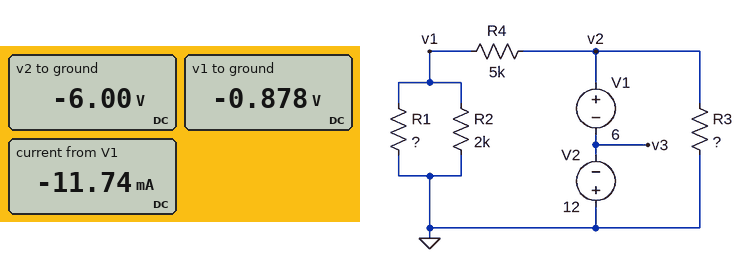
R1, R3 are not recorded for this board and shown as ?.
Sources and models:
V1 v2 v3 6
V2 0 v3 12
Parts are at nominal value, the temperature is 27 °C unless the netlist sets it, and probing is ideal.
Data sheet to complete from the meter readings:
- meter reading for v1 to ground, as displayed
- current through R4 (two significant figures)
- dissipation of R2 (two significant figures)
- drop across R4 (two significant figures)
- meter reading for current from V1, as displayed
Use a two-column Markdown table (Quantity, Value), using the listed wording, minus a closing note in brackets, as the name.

| Quantity | Value |
|---|---|
| meter reading for v1 to ground, as displayed | -0.878 V |
| current through R4 | 1.0 mA |
| dissipation of R2 | 390 µW |
| drop across R4 | 5.1 V |
| meter reading for current from V1, as displayed | -11.74 mA |
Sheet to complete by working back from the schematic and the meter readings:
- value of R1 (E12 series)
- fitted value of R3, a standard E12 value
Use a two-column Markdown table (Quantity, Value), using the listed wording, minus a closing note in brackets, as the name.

| Quantity | Value |
|---|---|
| value of R1 | 1.5 kΩ |
| fitted value of R3, a standard E12 value | 560 Ω |
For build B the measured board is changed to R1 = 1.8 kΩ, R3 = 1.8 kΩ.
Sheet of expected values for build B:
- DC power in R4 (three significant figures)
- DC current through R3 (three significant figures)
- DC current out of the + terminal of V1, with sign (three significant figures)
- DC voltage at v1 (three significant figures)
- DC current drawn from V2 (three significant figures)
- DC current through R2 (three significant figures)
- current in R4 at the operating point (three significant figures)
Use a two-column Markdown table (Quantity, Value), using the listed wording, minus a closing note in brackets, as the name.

| Quantity | Value |
|---|---|
| DC power in R4 | 5.09 mW |
| DC current through R3 | 3.33 mA |
| DC current out of the + terminal of V1, with sign | -4.34 mA |
| DC voltage at v1 | -956 mV |
| DC current drawn from V2 | 4.34 mA |
| DC current through R2 | 478 µA |
| current in R4 at the operating point | 1.01 mA |
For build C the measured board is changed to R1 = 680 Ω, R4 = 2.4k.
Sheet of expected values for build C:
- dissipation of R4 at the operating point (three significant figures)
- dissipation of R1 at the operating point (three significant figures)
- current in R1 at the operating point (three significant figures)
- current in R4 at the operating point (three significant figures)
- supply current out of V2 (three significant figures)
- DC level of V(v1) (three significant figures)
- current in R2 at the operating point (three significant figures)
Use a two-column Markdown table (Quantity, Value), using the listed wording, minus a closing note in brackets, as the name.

| Quantity | Value |
|---|---|
| dissipation of R4 at the operating point | 10.2 mW |
| dissipation of R1 at the operating point | 1.61 mW |
| current in R1 at the operating point | 1.54 mA |
| current in R4 at the operating point | 2.06 mA |
| supply current out of V2 | 12.8 mA |
| DC level of V(v1) | -1.05 V |
| current in R2 at the operating point | 524 µA |
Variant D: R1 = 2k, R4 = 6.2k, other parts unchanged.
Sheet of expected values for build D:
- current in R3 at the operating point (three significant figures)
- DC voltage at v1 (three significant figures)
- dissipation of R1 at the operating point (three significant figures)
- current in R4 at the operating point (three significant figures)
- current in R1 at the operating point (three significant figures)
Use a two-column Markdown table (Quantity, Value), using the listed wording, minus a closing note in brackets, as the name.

| Quantity | Value |
|---|---|
| current in R3 at the operating point | 10.7 mA |
| DC voltage at v1 | -833 mV |
| dissipation of R1 at the operating point | 347 µW |
| current in R4 at the operating point | 833 µA |
| current in R1 at the operating point | 417 µA |
